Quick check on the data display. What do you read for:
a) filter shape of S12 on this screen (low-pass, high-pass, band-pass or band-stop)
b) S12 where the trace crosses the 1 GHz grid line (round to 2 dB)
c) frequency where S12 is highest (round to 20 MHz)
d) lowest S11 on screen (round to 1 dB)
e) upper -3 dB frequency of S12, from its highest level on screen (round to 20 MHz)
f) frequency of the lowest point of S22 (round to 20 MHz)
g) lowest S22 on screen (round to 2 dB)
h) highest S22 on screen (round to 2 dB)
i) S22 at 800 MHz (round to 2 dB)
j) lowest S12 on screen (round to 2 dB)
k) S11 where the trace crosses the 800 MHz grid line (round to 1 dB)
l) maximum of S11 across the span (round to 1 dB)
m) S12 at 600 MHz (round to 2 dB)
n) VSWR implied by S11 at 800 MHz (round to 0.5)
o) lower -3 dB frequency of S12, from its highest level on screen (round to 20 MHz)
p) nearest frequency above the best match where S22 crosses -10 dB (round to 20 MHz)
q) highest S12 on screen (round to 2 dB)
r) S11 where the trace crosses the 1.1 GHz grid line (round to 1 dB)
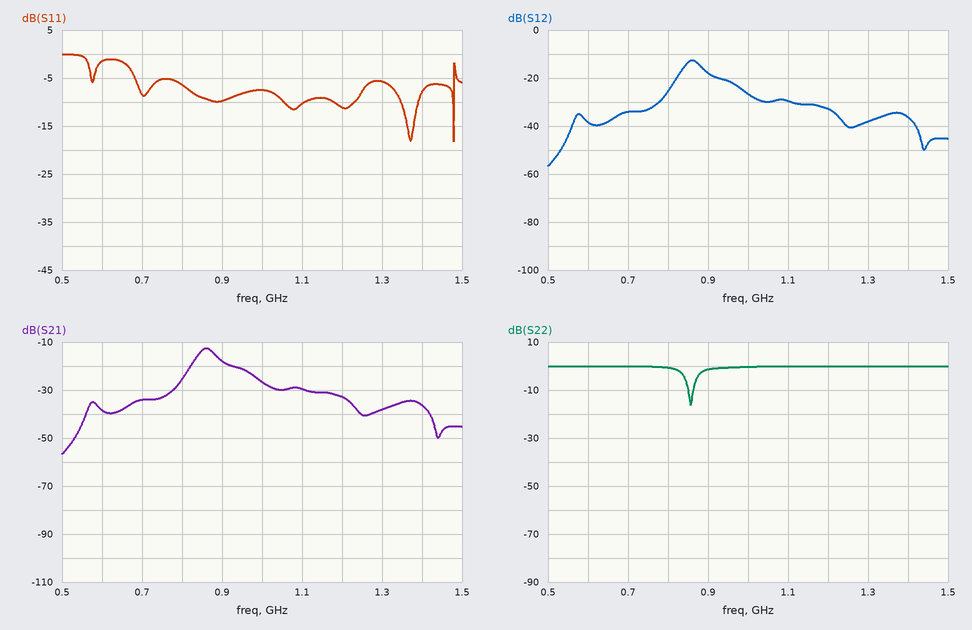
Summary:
band-pass
-26 dB
860 MHz
-18 dB
880 MHz
860 MHz
-16 dB
0 dB
0 dB
-56 dB
-6 dB
0 dB
-38 dB
3.0
840 MHz
860 MHz
-12 dB
-10 dB
